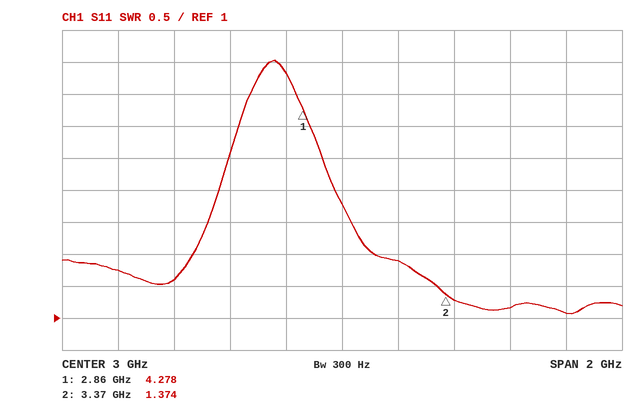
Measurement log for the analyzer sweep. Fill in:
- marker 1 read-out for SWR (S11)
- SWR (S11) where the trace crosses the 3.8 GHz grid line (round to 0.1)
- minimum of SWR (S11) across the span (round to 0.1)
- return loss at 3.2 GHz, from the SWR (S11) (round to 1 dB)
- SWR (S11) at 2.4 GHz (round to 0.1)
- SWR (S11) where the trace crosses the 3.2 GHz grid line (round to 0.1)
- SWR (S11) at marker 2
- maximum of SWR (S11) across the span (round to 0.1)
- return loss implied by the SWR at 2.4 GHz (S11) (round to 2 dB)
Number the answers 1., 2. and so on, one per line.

1. 4.278
2. 1.1
3. 1.1
4. 10 dB
5. 1.6
6. 1.9
7. 1.374
8. 5.0
9. 12 dB
